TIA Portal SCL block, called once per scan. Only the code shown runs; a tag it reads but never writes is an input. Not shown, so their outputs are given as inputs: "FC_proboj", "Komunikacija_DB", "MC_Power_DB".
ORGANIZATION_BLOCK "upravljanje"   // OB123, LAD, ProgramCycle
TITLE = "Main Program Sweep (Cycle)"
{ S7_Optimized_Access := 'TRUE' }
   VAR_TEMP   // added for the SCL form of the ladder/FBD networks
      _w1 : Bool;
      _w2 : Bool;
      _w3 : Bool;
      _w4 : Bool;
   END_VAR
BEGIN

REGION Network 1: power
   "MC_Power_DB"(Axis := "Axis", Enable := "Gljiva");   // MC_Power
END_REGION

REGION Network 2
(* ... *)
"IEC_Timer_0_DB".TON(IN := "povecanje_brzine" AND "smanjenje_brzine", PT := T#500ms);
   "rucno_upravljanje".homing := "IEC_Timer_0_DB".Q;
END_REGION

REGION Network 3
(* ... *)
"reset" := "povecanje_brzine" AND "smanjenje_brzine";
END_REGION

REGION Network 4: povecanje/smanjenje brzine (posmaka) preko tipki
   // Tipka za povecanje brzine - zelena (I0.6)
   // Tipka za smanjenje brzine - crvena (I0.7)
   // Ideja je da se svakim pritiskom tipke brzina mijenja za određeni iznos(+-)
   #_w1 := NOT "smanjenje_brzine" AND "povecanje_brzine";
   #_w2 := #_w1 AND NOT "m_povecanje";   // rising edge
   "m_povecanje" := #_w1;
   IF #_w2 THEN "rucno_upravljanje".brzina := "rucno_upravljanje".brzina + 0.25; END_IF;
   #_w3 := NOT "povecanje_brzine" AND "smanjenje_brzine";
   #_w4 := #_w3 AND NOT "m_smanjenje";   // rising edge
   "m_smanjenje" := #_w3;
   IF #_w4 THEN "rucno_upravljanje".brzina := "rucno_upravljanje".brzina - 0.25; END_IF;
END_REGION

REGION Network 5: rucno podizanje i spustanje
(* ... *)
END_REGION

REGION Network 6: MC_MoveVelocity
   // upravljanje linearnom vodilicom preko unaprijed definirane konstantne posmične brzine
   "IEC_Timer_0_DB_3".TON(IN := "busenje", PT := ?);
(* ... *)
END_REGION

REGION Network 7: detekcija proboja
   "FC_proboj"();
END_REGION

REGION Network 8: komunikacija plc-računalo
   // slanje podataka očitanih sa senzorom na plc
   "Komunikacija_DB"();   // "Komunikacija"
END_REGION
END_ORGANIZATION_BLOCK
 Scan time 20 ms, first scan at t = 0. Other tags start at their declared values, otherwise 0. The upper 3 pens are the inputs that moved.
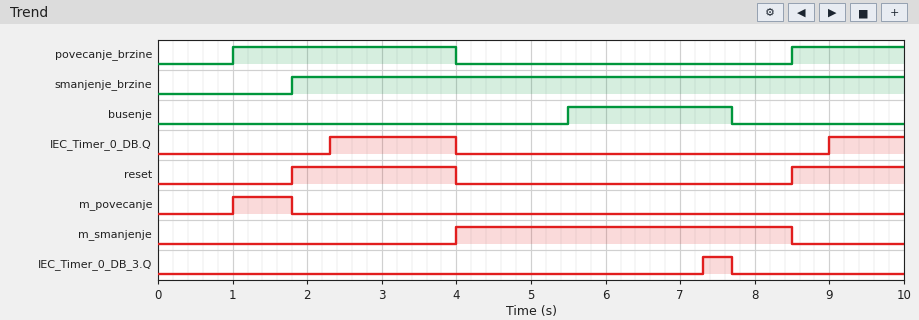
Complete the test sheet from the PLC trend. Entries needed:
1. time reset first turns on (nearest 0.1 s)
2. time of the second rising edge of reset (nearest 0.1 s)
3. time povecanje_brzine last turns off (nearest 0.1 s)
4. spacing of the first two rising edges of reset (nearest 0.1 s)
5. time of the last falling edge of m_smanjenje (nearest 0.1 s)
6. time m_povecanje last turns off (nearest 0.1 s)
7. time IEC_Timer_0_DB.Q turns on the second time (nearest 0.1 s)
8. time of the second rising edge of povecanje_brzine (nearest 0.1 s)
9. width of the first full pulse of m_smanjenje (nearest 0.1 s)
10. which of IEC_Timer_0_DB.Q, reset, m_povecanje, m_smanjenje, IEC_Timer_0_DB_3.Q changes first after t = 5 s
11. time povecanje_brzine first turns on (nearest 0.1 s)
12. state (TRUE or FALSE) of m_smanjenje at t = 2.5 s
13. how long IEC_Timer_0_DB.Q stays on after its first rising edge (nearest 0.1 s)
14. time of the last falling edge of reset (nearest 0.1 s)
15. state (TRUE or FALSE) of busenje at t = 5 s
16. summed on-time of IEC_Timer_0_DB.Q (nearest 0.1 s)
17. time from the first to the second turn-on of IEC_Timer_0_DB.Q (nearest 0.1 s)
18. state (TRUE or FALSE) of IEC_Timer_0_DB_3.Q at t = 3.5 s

1.8 s
8.5 s
4.0 s
6.7 s
8.5 s
1.8 s
9.0 s
8.5 s
4.5 s
IEC_Timer_0_DB_3.Q
1.0 s
FALSE
1.7 s
4.0 s
FALSE
2.7 s
6.7 s
FALSE
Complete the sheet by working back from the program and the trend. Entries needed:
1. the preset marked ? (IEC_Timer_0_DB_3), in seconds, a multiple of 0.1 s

1.8 s
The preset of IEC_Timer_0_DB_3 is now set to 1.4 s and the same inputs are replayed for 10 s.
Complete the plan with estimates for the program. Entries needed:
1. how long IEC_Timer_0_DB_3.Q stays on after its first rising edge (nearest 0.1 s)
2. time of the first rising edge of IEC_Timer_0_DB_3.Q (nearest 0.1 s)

0.8 s
6.9 s
